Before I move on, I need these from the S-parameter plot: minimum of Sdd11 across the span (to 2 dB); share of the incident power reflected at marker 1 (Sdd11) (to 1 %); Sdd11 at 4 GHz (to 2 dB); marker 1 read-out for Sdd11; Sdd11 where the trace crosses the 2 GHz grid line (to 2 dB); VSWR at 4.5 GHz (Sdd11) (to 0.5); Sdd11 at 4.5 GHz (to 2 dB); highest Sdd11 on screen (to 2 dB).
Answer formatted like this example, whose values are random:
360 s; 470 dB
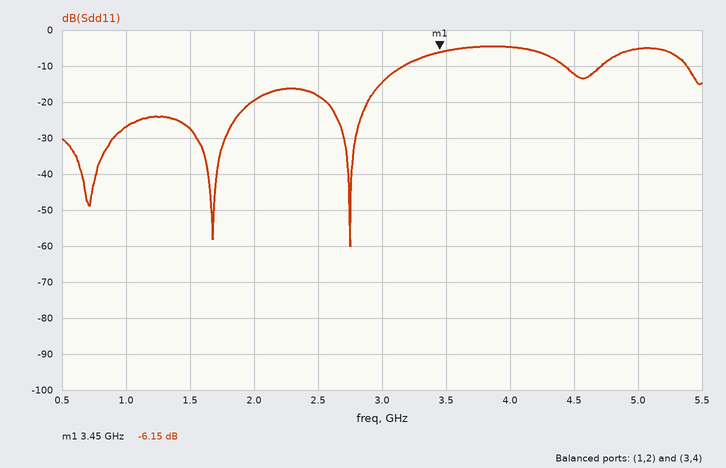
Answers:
-60 dB; 24 %; -4 dB; -6.15 dB; -20 dB; 1.5; -12 dB; -4 dB
